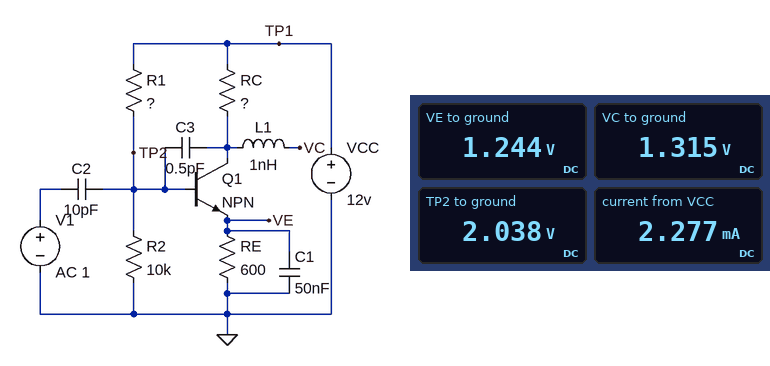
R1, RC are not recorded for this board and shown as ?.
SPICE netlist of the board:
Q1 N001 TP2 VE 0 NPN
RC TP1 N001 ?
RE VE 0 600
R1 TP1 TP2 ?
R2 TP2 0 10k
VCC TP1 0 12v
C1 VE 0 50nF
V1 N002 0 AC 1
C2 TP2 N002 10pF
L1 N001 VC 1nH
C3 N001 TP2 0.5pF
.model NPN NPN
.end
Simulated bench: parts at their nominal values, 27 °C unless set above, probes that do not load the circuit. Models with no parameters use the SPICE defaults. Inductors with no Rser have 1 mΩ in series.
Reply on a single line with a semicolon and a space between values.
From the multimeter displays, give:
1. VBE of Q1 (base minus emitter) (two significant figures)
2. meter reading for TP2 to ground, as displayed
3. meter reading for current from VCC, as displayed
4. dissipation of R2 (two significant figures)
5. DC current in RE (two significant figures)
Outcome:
790 mV; 2.038 V; 2.277 mA; 420 µW; 2.1 mA
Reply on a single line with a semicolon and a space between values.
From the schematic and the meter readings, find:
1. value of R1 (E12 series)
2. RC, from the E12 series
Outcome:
27 kΩ; 5.6 kΩ
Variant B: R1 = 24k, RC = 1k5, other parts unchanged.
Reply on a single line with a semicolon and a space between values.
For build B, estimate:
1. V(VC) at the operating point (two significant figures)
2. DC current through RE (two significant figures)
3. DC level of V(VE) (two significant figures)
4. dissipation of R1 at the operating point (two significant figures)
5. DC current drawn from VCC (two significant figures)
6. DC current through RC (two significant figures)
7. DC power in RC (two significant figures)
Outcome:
6.0 V; 4.1 mA; 2.4 V; 3.2 mW; 4.4 mA; 4.0 mA; 24 mW
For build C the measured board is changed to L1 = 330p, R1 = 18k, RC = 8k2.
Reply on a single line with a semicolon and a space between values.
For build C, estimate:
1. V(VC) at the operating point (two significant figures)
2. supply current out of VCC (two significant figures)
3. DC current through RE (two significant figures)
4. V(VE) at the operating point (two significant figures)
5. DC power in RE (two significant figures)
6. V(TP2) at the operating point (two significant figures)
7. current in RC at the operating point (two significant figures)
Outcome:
1.1 V; 1.9 mA; 1.7 mA; 1.0 V; 1.8 mW; 1.8 V; 1.3 mA
